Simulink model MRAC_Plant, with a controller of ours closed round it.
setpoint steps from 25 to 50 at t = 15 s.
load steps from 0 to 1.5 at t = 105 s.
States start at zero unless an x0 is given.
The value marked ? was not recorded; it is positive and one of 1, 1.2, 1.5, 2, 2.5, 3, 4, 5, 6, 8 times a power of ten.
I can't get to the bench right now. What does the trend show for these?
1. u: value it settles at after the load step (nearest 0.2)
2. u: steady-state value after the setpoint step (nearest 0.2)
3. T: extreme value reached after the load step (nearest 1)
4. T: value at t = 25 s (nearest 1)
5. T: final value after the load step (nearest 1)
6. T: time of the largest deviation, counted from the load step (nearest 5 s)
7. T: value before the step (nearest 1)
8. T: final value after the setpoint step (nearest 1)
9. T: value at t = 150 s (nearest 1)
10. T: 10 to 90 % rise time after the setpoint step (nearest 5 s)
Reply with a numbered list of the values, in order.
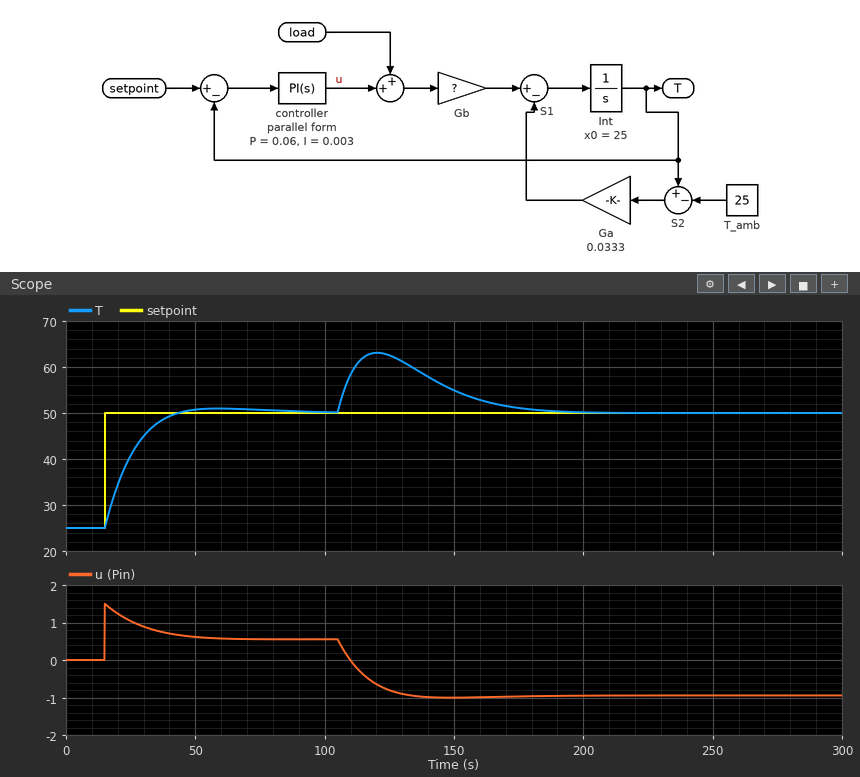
1. -1.0
2. 0.6
3. 63
4. 41
5. 50
6. 15 s
7. 25
8. 50
9. 55
10. 20 s
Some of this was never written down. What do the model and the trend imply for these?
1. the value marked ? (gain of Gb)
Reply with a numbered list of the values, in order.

1. 1.5
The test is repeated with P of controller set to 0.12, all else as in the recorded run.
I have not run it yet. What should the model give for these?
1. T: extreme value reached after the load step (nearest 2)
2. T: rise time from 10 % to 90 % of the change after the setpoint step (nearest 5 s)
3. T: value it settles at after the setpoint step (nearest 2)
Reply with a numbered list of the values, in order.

1. 58
2. 15 s
3. 50
